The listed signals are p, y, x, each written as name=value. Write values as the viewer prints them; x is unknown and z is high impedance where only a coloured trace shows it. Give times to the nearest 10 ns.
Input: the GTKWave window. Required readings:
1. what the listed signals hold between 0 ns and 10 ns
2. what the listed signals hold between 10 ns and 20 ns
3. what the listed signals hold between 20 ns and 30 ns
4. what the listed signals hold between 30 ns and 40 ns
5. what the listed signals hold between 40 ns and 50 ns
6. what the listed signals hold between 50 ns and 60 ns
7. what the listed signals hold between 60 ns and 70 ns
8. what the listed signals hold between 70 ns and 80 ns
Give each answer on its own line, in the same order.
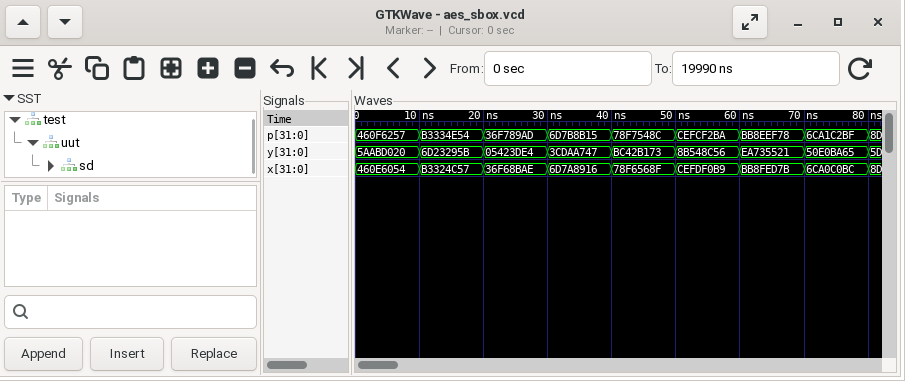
p=460F6257, y=5AABD020, x=460E6054
p=B3334E54, y=6D23295B, x=B3324C57
p=36F789AD, y=05423DE4, x=36F68BAE
p=6D7B8B15, y=3CDAA747, x=6D7A8916
p=78F7548C, y=BC42B173, x=78F6568F
p=CEFCF2BA, y=8B548C56, x=CEFDF0B9
p=BB8EEF78, y=EA735521, x=BB8FED7B
p=6CA1C2BF, y=50E0BA65, x=6CA0C0BC
